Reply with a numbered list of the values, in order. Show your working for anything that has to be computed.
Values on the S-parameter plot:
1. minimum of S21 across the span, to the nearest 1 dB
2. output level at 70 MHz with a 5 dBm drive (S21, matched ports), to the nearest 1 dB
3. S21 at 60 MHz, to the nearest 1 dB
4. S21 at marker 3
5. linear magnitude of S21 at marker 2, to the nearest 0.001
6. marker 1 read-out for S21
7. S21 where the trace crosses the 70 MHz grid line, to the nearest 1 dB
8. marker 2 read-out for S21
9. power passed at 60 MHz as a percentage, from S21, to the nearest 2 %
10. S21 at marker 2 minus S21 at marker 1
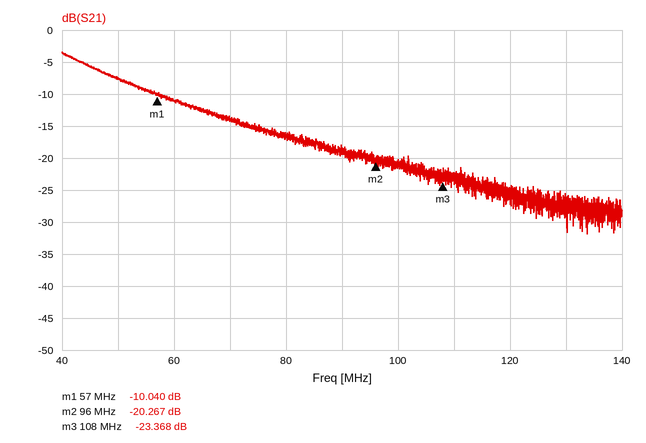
1. -32 dB
2. 5 dBm + (-14 dB) = -9 dBm
3. -11 dB
4. -23.368 dB
5. 10^(-20.267/20) ≈ 0.097
6. -10.040 dB
7. -14 dB
8. -20.267 dB
9. 10^(-11/10) ≈ 8 %
10. -20.267 − (-10.04) = -10.227 dB
